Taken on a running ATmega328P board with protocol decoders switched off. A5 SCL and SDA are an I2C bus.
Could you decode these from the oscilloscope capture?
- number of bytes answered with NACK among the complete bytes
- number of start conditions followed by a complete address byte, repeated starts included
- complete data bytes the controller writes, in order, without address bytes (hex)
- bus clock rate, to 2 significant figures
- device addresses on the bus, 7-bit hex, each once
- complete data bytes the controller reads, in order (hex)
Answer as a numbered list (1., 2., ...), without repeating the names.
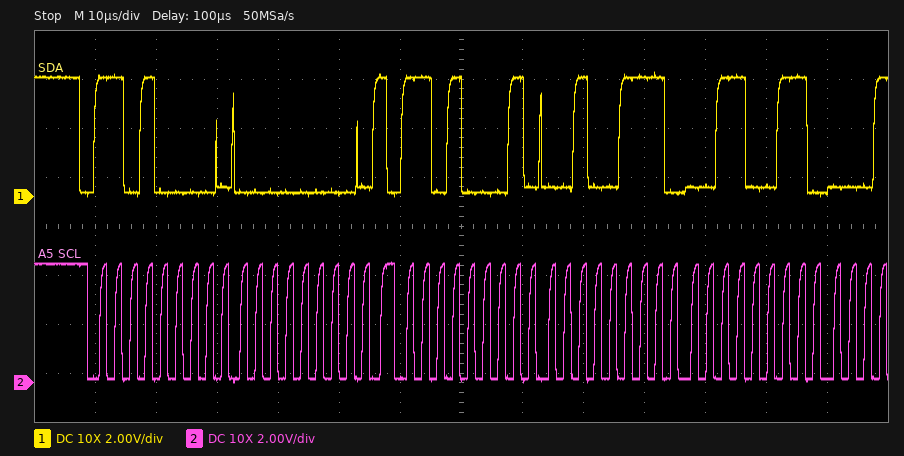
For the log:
1. 0
2. 2
3. 00
4. 400 kHz
5. 0x68
6. 27 33
